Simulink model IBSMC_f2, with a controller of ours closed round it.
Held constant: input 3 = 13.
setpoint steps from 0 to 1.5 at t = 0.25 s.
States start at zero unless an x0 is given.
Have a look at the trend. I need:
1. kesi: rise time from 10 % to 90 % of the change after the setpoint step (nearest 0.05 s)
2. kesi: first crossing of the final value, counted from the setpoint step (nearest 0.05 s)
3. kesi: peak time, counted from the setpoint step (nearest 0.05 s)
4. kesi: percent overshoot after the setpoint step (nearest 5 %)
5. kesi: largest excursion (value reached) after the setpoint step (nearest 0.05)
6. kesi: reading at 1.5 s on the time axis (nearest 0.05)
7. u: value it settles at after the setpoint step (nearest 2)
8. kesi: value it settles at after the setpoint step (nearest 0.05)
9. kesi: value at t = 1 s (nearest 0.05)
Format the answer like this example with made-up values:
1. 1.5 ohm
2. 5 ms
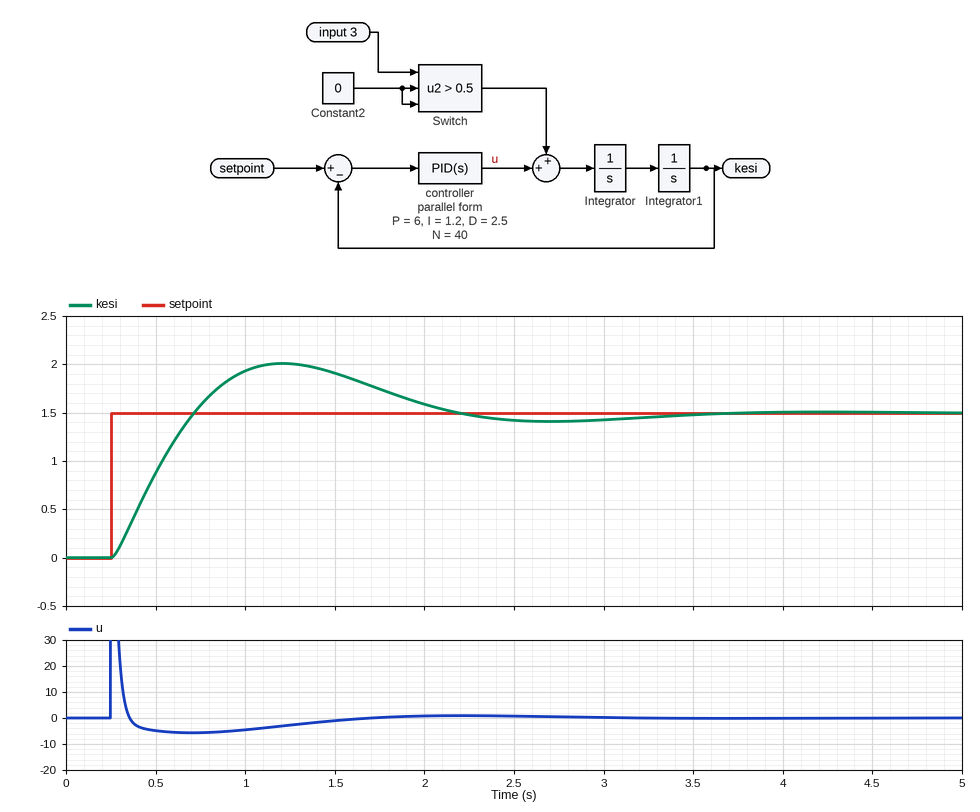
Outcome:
1. 0.35 s
2. 0.45 s
3. 0.95 s
4. 35 %
5. 2.00
6. 1.90
7. 0
8. 1.50
9. 1.95
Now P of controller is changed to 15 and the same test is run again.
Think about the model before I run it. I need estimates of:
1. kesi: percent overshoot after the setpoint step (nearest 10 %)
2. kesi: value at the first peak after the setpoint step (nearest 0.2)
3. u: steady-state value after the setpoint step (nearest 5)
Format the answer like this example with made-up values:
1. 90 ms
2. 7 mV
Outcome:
1. 50 %
2. 2.2
3. 0
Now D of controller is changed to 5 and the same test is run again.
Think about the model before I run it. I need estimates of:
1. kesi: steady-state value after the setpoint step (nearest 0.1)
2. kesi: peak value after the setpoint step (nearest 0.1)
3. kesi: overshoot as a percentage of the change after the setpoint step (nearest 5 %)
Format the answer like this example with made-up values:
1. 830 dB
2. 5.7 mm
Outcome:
1. 1.5
2. 1.7
3. 15 %
